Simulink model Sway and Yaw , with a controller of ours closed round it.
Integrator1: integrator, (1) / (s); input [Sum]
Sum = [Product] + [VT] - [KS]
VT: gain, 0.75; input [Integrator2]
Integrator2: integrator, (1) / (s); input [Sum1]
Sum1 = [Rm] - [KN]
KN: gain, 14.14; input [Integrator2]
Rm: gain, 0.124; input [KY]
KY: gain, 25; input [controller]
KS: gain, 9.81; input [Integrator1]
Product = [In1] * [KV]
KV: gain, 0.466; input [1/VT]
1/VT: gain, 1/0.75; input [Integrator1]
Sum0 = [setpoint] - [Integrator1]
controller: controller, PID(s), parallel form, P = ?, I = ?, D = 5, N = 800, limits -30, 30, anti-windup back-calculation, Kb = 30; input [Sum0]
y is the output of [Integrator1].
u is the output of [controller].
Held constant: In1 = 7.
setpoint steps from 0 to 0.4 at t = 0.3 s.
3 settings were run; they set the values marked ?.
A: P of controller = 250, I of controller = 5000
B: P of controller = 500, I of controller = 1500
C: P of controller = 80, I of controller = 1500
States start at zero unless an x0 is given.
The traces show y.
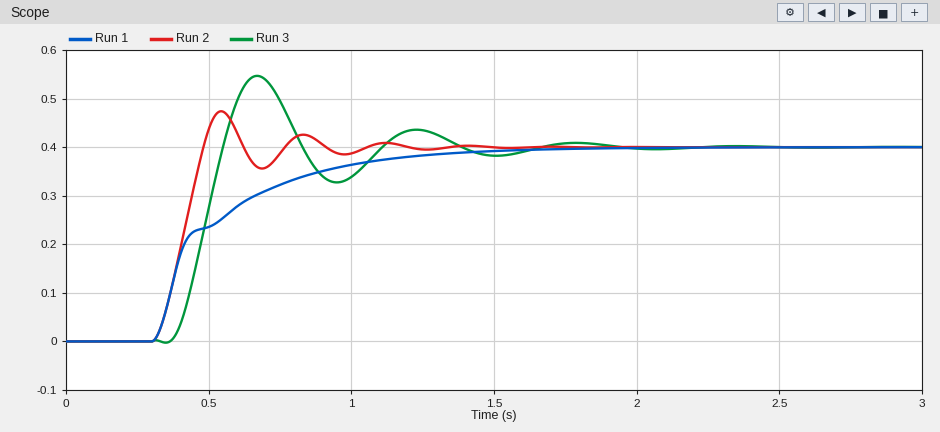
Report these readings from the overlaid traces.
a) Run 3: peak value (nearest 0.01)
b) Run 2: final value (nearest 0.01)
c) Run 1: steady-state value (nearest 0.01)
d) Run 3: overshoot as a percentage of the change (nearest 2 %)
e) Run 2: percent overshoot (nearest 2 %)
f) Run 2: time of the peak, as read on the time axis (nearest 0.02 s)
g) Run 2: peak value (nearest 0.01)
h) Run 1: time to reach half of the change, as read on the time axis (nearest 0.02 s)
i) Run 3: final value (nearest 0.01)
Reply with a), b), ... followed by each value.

a) 0.55
b) 0.40
c) 0.40
d) 36 %
e) 18 %
f) 0.54 s
g) 0.47
h) 0.42 s
i) 0.40
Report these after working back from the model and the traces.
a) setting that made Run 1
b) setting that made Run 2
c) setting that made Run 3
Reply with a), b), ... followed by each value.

a) B
b) A
c) C
